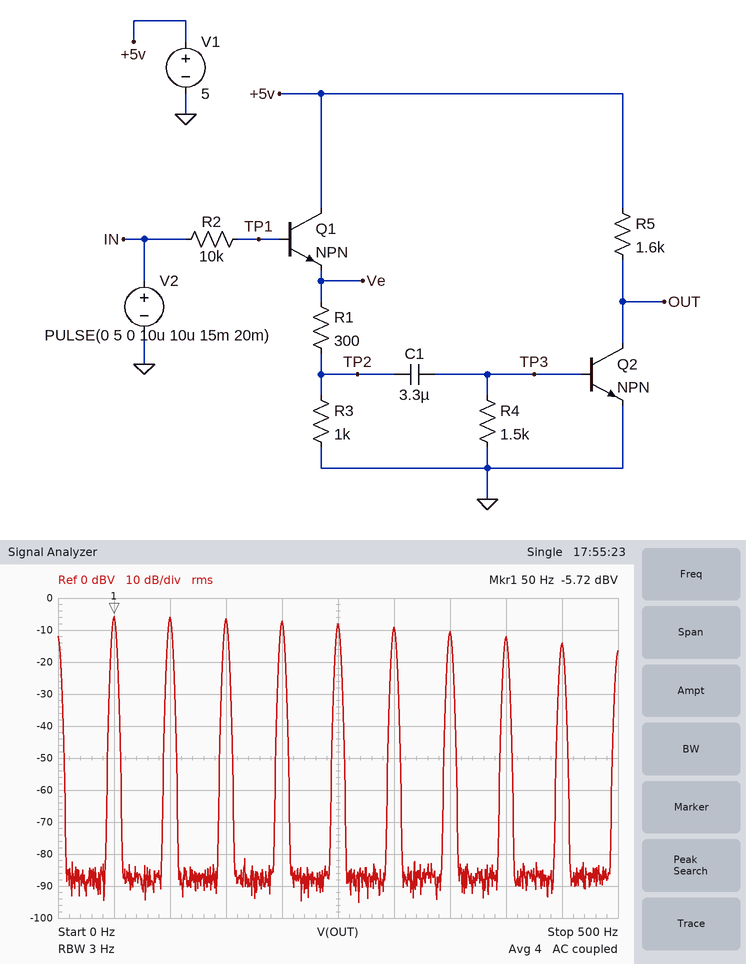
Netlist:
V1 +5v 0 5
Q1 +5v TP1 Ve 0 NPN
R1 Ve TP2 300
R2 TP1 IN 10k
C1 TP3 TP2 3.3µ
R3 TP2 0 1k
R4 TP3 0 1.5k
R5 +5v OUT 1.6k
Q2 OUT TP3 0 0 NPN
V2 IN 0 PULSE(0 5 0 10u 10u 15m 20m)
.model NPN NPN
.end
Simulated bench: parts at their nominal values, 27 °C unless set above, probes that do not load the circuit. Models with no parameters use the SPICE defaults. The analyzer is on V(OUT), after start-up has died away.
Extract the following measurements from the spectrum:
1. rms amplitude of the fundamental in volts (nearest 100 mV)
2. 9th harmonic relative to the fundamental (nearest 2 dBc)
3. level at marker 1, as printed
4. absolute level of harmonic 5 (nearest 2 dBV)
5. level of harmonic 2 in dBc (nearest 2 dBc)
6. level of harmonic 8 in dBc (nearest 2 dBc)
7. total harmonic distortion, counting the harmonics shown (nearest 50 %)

500 mV
-8 dBc
-5.72 dBV
-8 dBV
0 dBc
-6 dBc
200 %
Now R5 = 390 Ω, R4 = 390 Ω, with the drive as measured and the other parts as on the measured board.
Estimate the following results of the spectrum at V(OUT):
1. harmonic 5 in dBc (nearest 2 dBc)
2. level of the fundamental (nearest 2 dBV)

0 dBc
-14 dBV
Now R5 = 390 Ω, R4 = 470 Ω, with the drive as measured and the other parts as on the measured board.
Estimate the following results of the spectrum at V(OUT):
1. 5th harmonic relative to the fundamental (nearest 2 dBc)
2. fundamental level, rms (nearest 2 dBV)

0 dBc
-12 dBV
